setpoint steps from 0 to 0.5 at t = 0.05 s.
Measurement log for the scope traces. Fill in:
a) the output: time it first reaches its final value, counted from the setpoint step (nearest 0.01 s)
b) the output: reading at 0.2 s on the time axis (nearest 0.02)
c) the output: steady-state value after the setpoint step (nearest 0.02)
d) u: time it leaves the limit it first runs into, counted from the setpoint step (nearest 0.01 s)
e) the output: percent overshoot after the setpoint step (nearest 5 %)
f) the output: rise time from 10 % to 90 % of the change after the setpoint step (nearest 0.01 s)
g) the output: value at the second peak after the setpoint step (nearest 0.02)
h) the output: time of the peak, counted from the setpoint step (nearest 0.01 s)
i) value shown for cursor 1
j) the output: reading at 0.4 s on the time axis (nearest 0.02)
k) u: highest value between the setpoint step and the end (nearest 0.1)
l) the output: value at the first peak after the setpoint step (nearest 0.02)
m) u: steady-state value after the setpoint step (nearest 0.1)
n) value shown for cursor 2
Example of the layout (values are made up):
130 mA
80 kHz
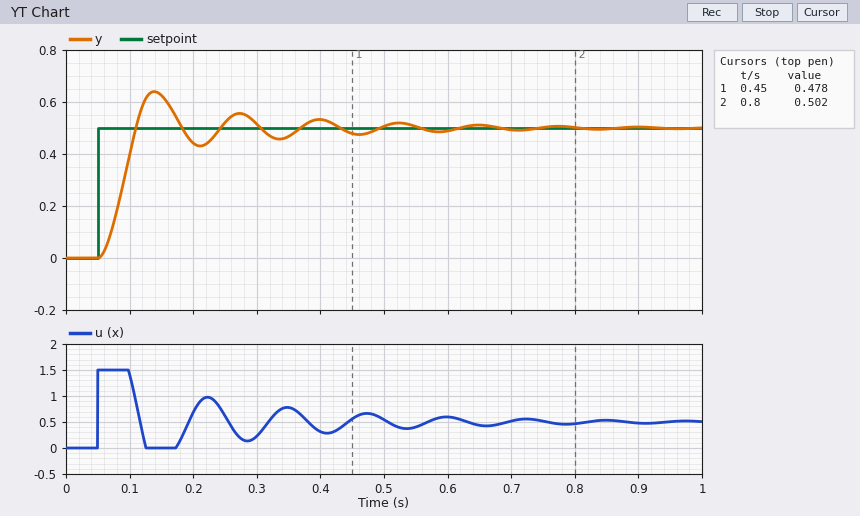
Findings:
0.06 s
0.44
0.50
0.05 s
30 %
0.04 s
0.56
0.09 s
0.478
0.54
1.5
0.64
0.5
0.502
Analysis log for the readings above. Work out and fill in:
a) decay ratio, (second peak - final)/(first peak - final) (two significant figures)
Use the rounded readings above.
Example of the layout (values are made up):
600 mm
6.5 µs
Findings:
0.43
